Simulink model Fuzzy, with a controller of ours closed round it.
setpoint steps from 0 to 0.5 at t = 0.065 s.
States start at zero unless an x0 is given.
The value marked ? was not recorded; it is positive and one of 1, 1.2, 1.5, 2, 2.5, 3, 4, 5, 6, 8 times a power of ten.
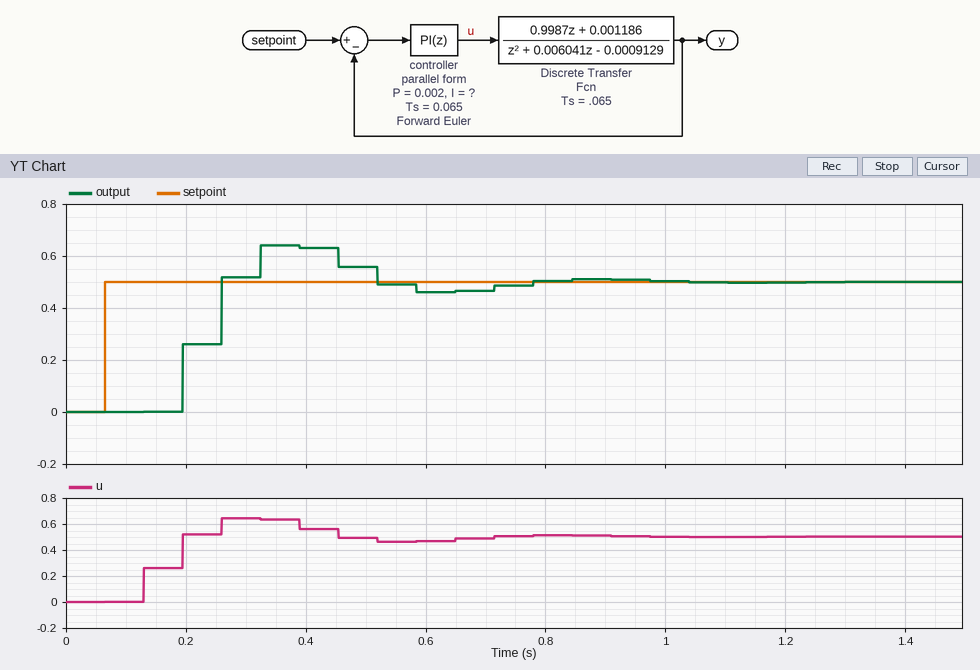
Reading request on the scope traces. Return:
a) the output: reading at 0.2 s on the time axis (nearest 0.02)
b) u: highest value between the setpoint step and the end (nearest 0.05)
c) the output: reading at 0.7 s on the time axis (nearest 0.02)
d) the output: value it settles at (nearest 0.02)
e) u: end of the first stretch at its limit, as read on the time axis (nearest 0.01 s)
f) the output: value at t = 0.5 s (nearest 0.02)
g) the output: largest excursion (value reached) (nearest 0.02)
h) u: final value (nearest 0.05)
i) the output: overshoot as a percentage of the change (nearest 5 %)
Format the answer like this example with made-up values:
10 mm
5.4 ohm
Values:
0.26
0.65
0.46
0.50
0.13 s
0.56
0.64
0.50
30 %
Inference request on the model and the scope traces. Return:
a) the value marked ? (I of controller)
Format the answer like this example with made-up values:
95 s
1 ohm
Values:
8
